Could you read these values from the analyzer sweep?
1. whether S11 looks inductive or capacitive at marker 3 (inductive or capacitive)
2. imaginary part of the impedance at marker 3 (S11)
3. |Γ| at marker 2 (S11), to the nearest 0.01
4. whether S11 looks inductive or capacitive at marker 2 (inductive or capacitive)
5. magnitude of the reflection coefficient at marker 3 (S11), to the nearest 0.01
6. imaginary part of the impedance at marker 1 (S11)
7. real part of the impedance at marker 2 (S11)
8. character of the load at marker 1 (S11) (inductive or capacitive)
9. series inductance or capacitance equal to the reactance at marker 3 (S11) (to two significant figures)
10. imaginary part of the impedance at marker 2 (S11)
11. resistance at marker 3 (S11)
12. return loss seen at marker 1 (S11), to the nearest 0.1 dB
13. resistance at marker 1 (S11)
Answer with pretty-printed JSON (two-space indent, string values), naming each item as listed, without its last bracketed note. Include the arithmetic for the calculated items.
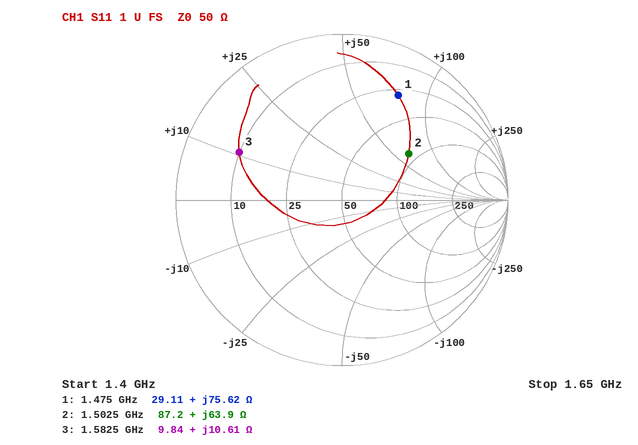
{
  "whether S11 looks inductive or capacitive at marker 3": "inductive",
  "imaginary part of the impedance at marker 3": "+10.61 Ω",
  "|Γ| at marker 2 (S11), to the nearest 0.01": "0.49",
  "whether S11 looks inductive or capacitive at marker 2": "inductive",
  "magnitude of the reflection coefficient at marker 3 (S11), to the nearest 0.01": "0.68",
  "imaginary part of the impedance at marker 1": "+75.62 Ω",
  "real part of the impedance at marker 2": "87.2 Ω",
  "character of the load at marker 1 (S11)": "inductive",
  "series inductance or capacitance equal to the reactance at marker 3 (S11)": "L = 10.61 Ω/(2π × 1.5825 GHz) ≈ 1.1 nH",
  "imaginary part of the impedance at marker 2": "+63.9 Ω",
  "resistance at marker 3": "9.84 Ω",
  "return loss seen at marker 1 (S11), to the nearest 0.1 dB": "2.9 dB",
  "resistance at marker 1": "29.11 Ω"
}
